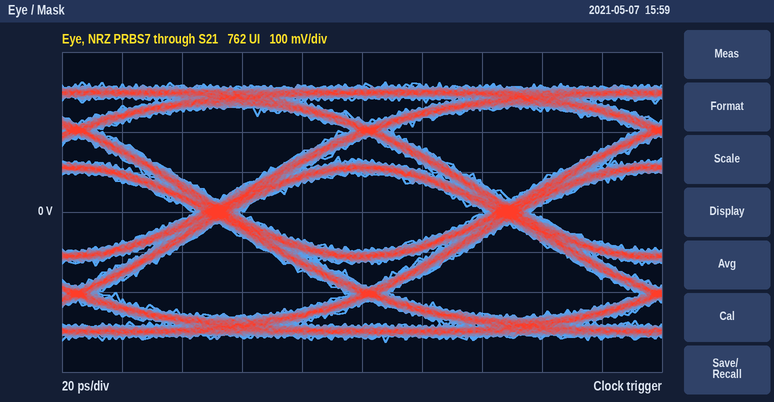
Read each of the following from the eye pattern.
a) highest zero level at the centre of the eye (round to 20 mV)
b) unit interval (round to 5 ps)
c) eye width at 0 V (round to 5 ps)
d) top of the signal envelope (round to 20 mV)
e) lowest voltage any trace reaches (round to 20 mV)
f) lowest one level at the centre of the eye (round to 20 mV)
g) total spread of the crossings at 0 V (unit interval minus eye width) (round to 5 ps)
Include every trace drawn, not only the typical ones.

-100 mV
95 ps
80 ps
320 mV
-320 mV
100 mV
15 ps
